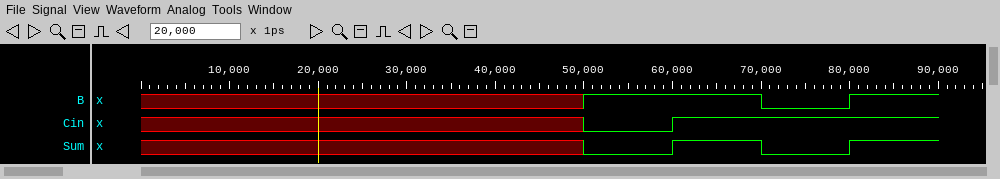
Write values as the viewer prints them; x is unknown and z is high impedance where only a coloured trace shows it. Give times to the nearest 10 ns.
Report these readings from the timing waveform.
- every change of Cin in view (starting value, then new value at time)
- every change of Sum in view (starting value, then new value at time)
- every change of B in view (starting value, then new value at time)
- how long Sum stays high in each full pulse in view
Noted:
x, 0 at 50 ns, 1 at 60 ns
x, 0 at 50 ns, 1 at 60 ns, 0 at 70 ns, 1 at 80 ns
x, 1 at 50 ns, 0 at 70 ns, 1 at 80 ns
10 ns
